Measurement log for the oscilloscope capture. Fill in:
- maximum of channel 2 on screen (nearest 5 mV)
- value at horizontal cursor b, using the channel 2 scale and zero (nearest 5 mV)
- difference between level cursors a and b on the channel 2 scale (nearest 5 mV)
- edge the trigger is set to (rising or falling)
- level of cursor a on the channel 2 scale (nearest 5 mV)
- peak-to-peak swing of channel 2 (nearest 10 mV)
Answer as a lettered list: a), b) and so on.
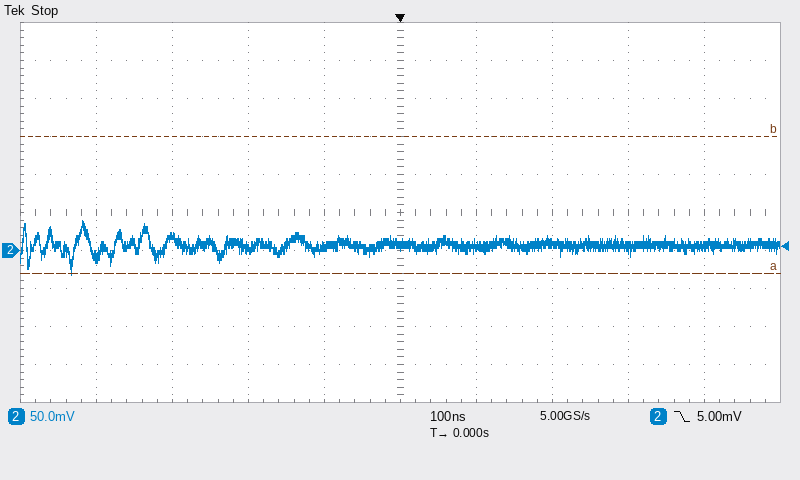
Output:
a) 40 mV
b) 150 mV
c) 180 mV
d) falling
e) -30 mV
f) 70 mV
